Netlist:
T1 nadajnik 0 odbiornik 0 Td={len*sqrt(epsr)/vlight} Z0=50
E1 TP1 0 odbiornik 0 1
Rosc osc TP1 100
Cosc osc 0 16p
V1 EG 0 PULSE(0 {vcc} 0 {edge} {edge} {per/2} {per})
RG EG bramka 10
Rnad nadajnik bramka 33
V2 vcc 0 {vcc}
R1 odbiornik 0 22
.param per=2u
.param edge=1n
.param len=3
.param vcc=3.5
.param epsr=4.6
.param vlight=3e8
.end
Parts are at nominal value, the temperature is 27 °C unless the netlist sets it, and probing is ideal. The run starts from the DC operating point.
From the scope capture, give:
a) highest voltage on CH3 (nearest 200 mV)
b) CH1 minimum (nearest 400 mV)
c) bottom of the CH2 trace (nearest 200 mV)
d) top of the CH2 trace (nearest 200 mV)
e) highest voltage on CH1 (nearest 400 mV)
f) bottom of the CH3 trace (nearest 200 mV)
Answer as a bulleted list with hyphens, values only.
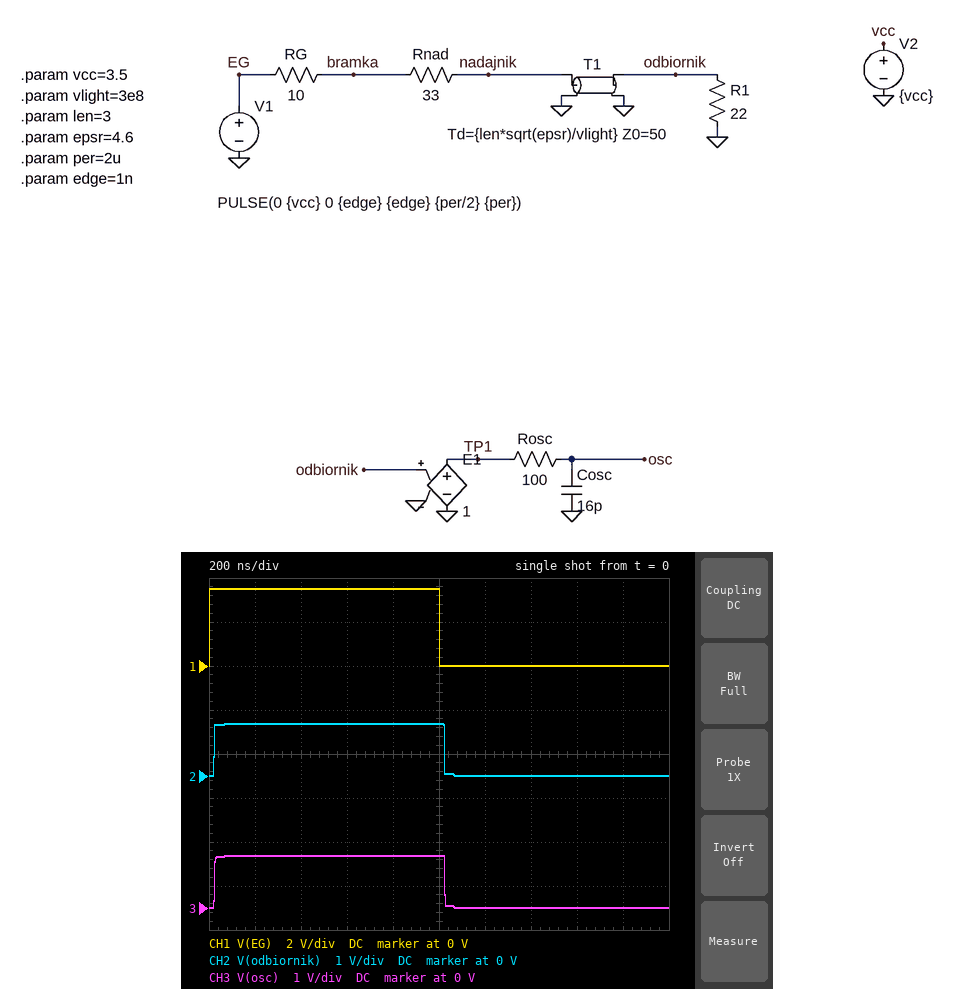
- 1.2 V
- 0 V
- 0 V
- 1.2 V
- 3.6 V
- 0 V
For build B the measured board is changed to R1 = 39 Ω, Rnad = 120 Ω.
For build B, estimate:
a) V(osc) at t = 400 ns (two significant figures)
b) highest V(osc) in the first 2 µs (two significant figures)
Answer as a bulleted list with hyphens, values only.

- 810 mV
- 850 mV
